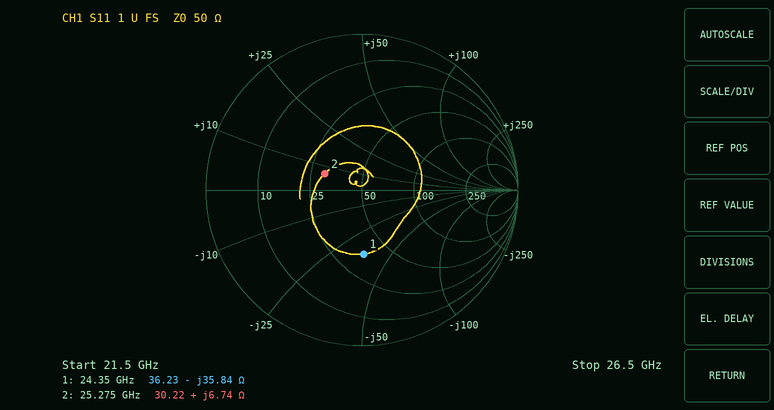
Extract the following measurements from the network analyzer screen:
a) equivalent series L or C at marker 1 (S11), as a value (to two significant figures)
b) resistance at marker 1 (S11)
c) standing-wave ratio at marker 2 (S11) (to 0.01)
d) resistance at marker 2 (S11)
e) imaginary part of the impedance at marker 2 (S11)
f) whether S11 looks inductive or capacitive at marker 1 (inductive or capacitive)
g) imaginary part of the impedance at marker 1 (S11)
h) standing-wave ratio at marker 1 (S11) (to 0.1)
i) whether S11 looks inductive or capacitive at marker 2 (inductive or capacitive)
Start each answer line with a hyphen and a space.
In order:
- 180 fF
- 36.23 Ω
- 1.70
- 30.22 Ω
- +6.74 Ω
- capacitive
- -35.84 Ω
- 2.4
- inductive
